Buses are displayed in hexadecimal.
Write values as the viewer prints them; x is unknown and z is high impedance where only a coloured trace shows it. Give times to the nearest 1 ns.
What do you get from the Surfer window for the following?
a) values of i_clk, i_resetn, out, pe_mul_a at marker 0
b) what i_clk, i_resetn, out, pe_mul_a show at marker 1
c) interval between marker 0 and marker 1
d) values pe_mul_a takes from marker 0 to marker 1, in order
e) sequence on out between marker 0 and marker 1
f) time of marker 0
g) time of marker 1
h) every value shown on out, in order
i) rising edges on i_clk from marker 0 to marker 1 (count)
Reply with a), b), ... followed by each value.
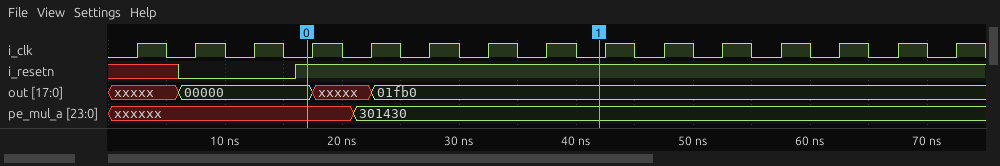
a) i_clk=0, i_resetn=1, out=00000, pe_mul_a=xxxxxx
b) i_clk=0, i_resetn=1, out=01fb0, pe_mul_a=301430
c) 25 ns
d) xxxxxx, 301430
e) 00000, xxxxx, 01fb0
f) 17 ns
g) 42 ns
h) xxxxx, 00000, xxxxx, 01fb0
i) 5
